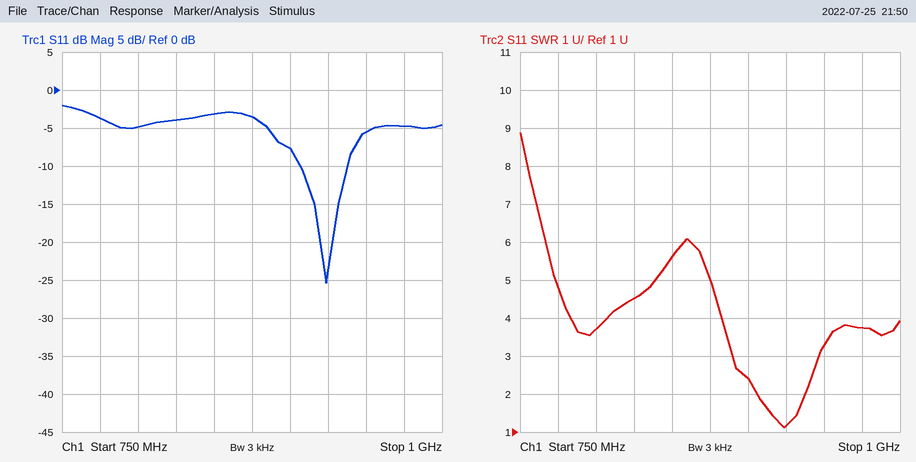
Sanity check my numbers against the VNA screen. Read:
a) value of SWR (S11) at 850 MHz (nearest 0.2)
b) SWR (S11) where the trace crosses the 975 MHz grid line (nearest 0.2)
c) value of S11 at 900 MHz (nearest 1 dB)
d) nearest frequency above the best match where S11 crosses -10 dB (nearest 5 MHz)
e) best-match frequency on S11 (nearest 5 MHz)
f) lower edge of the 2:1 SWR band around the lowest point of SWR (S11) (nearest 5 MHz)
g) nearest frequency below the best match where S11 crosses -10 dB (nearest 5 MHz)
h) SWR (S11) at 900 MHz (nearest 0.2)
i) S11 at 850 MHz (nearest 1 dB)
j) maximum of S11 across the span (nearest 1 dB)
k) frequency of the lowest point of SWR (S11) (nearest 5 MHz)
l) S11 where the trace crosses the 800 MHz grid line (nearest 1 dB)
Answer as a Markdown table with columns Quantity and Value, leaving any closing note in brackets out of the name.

| Quantity | Value |
|---|---|
| value of SWR (S11) at 850 MHz | 5.6 |
| SWR (S11) where the trace crosses the 975 MHz grid line | 3.8 |
| value of S11 at 900 MHz | -8 dB |
| nearest frequency above the best match where S11 crosses -10 dB | 940 MHz |
| best-match frequency on S11 | 925 MHz |
| lower edge of the 2:1 SWR band around the lowest point of SWR (S11) | 905 MHz |
| nearest frequency below the best match where S11 crosses -10 dB | 905 MHz |
| SWR (S11) at 900 MHz | 2.4 |
| S11 at 850 MHz | -3 dB |
| maximum of S11 across the span | -2 dB |
| frequency of the lowest point of SWR (S11) | 925 MHz |
| S11 where the trace crosses the 800 MHz grid line | -5 dB |
